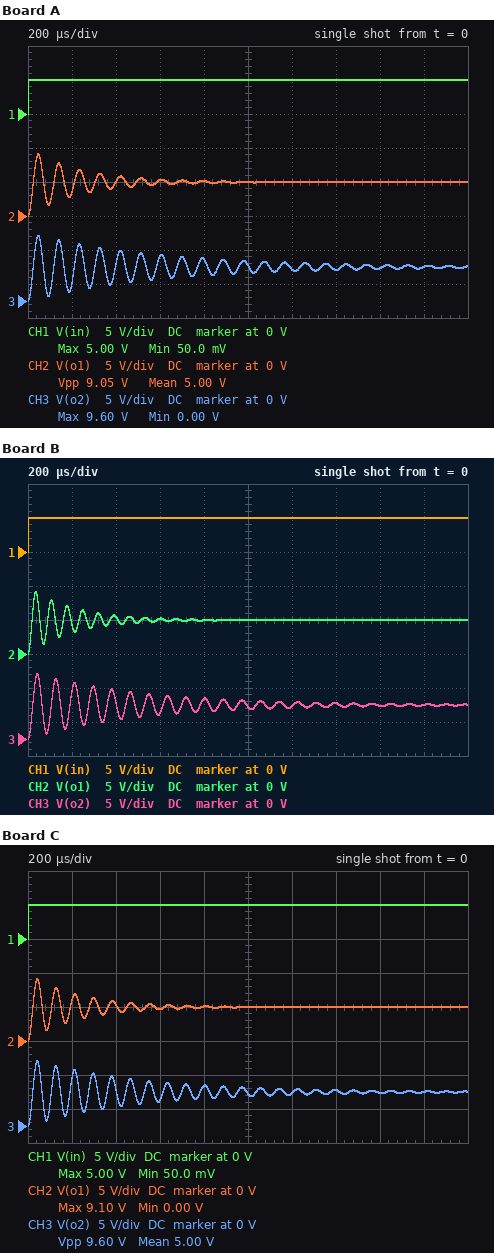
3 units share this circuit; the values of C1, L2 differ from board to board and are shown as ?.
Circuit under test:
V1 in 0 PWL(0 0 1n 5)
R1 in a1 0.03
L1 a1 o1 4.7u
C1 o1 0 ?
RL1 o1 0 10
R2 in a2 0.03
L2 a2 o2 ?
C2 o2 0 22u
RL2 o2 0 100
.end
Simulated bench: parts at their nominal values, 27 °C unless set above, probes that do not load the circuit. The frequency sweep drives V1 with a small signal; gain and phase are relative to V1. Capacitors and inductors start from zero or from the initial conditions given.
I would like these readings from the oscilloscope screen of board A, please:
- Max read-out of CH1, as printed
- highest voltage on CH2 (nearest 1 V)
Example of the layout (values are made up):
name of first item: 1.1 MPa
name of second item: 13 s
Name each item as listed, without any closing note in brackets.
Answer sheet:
Max read-out of CH1, as printed: 5.00 V
highest voltage on CH2: 9 V
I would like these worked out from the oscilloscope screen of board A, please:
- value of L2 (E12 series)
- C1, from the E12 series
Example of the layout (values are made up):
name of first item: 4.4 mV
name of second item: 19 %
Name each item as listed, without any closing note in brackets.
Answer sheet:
value of L2: 10 µH
C1, from the E12 series: 47 µF
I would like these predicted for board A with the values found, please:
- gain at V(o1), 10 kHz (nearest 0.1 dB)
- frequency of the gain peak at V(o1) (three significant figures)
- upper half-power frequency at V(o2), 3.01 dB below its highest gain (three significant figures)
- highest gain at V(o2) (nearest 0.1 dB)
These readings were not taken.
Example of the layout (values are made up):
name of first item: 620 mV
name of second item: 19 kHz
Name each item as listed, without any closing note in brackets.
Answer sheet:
gain at V(o1), 10 kHz: 15.1 dB
frequency of the gain peak at V(o1): 10.7 kHz
upper half-power frequency at V(o2), 3.01 dB below its highest gain: 11.0 kHz
highest gain at V(o2): 25.8 dB
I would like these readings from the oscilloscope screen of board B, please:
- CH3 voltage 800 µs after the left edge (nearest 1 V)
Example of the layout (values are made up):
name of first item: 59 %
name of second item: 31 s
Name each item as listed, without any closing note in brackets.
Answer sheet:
CH3 voltage 800 µs after the left edge: 6 V
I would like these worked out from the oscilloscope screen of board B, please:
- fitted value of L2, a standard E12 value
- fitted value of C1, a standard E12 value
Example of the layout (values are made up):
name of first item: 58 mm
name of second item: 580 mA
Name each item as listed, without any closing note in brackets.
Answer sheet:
fitted value of L2, a standard E12 value: 8.2 µH
fitted value of C1, a standard E12 value: 27 µF
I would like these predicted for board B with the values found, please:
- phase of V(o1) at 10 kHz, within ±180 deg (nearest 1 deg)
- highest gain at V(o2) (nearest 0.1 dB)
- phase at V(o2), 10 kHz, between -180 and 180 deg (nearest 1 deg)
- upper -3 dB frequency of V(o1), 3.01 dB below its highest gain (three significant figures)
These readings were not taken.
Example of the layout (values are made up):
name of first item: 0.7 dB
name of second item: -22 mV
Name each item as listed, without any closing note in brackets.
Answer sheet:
phase of V(o1) at 10 kHz, within ±180 deg: -9 deg
highest gain at V(o2): 25.2 dB
phase at V(o2), 10 kHz, between -180 and 180 deg: -9 deg
upper -3 dB frequency of V(o1), 3.01 dB below its highest gain: 14.9 kHz
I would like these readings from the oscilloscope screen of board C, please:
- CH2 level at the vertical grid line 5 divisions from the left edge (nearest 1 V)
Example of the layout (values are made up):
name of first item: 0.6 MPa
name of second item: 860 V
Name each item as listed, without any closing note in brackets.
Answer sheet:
CH2 level at the vertical grid line 5 divisions from the left edge: 5 V
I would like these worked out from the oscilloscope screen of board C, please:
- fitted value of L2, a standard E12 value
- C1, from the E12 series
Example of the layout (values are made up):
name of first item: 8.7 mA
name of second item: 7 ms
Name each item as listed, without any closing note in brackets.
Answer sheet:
fitted value of L2, a standard E12 value: 8.2 µH
C1, from the E12 series: 39 µF
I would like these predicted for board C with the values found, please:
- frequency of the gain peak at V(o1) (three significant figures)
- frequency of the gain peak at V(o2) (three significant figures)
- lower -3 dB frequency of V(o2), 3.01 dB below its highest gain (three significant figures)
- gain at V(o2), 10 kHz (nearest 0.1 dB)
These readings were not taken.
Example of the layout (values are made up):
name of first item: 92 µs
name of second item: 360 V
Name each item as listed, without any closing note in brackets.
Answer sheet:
frequency of the gain peak at V(o1): 11.7 kHz
frequency of the gain peak at V(o2): 11.8 kHz
lower -3 dB frequency of V(o2), 3.01 dB below its highest gain: 11.5 kHz
gain at V(o2), 10 kHz: 10.7 dB
